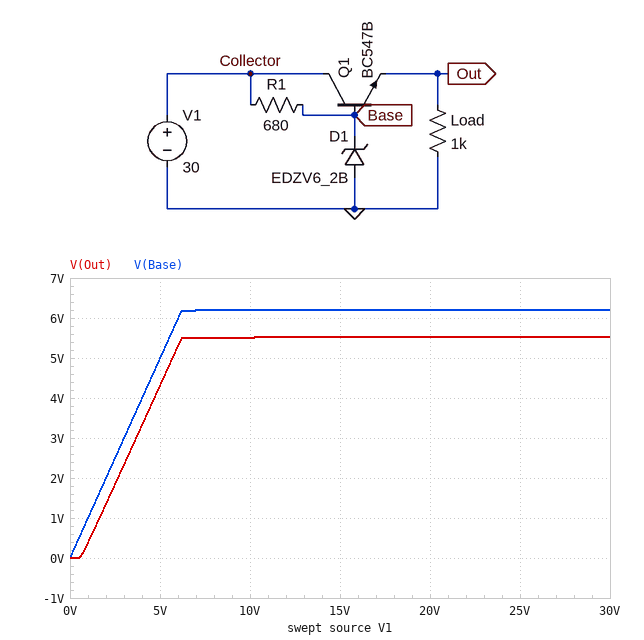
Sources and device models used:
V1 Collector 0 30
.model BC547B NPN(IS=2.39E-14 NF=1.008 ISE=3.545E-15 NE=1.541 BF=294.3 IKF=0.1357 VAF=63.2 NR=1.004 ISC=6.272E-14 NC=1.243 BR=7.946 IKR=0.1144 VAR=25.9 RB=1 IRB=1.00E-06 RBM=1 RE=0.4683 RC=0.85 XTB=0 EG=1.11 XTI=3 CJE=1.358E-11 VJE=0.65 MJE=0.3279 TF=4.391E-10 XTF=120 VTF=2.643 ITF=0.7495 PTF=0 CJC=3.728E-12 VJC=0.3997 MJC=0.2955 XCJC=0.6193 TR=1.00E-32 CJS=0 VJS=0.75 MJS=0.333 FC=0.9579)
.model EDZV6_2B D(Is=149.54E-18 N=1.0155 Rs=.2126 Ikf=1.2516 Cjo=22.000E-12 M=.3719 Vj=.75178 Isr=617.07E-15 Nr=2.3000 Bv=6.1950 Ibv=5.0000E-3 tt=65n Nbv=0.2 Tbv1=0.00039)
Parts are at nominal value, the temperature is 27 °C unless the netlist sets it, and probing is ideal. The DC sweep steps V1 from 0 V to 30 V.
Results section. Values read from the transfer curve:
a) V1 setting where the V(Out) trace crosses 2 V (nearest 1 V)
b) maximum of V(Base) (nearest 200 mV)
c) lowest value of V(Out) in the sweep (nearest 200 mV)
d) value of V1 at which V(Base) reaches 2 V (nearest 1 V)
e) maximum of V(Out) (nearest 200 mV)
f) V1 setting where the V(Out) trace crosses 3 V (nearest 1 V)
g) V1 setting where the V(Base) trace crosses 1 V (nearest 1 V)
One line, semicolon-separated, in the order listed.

3 V; 6.2 V; 0 V; 2 V; 5.6 V; 4 V; 1 V
